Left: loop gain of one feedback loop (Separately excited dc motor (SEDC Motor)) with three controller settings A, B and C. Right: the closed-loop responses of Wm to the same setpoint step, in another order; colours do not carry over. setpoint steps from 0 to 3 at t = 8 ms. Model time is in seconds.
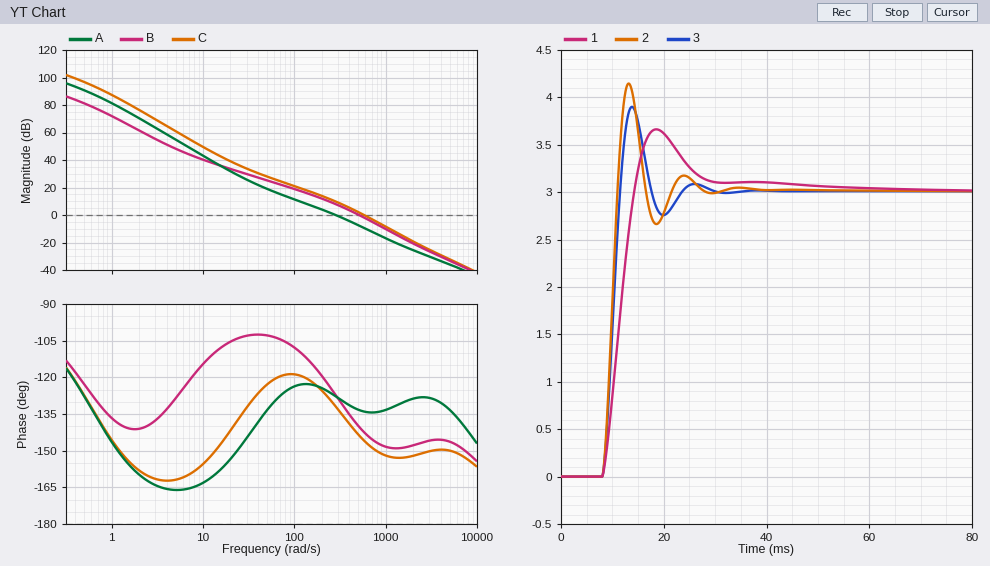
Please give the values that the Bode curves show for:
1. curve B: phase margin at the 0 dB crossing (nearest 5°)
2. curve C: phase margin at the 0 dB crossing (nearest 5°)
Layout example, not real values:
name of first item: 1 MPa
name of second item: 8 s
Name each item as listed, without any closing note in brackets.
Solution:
curve B: phase margin at the 0 dB crossing: 40°
curve C: phase margin at the 0 dB crossing: 35°
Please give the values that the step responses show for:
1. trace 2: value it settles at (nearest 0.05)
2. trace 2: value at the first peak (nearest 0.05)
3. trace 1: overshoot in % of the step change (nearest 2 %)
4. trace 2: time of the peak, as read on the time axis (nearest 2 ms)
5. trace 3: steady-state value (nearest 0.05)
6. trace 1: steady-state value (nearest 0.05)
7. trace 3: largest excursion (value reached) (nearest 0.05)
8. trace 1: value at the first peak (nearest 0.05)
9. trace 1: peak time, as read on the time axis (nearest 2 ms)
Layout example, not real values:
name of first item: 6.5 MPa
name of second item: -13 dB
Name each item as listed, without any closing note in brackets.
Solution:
trace 2: value it settles at: 3.00
trace 2: value at the first peak: 4.15
trace 1: overshoot in % of the step change: 22 %
trace 2: time of the peak, as read on the time axis: 14 ms
trace 3: steady-state value: 3.00
trace 1: steady-state value: 3.00
trace 3: largest excursion (value reached): 3.90
trace 1: value at the first peak: 3.65
trace 1: peak time, as read on the time axis: 18 ms
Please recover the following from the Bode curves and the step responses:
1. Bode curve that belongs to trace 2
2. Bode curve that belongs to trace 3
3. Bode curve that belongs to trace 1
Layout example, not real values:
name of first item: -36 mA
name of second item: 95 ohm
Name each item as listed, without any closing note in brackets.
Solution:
Bode curve that belongs to trace 2: C
Bode curve that belongs to trace 3: B
Bode curve that belongs to trace 1: A
